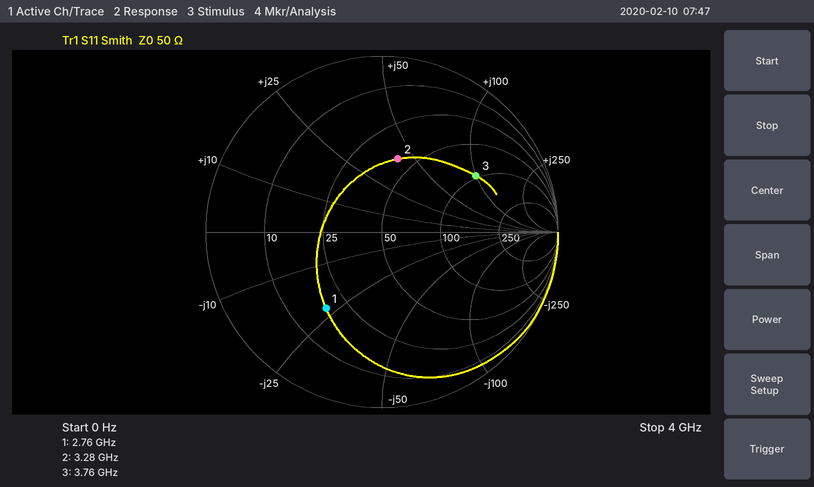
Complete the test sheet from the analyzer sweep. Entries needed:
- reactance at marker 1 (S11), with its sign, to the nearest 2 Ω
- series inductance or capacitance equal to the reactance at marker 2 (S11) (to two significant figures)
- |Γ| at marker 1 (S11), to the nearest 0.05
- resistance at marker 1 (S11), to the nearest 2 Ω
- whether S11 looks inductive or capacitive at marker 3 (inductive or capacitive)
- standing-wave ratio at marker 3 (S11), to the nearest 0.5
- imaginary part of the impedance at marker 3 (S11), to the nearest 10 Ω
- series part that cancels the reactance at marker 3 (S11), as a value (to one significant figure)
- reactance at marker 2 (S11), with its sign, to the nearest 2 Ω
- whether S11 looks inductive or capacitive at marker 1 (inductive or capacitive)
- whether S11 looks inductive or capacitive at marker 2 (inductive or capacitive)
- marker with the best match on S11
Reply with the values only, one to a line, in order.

-22 Ω
2.0 nH
0.55
18 Ω
inductive
4.5
+100 Ω
400 fF
+42 Ω
capacitive
inductive
marker 2
